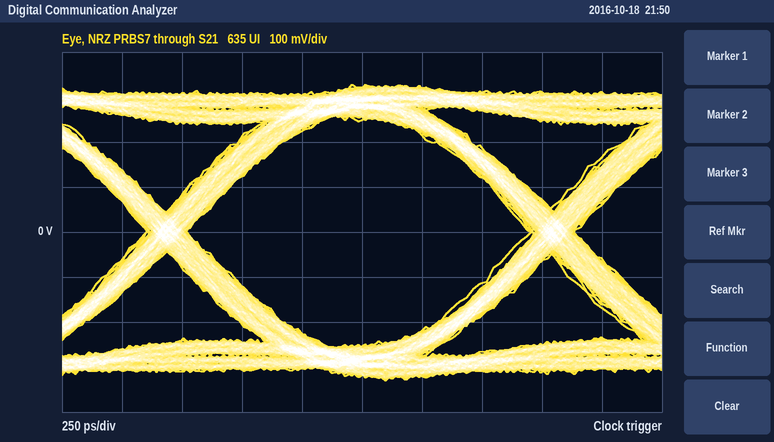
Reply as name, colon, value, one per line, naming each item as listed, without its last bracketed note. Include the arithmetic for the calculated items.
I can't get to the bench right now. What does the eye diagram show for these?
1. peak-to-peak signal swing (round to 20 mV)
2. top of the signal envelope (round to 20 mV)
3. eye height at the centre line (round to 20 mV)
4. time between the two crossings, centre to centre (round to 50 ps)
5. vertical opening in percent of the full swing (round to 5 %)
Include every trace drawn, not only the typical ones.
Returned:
peak-to-peak signal swing: 660 mV
top of the signal envelope: 320 mV
eye height at the centre line: 500 mV
time between the two crossings, centre to centre: 1.60 ns
vertical opening in percent of the full swing: 500 mV / 660 mV ≈ 75.8 %, so 75 % to the nearest 5 %
